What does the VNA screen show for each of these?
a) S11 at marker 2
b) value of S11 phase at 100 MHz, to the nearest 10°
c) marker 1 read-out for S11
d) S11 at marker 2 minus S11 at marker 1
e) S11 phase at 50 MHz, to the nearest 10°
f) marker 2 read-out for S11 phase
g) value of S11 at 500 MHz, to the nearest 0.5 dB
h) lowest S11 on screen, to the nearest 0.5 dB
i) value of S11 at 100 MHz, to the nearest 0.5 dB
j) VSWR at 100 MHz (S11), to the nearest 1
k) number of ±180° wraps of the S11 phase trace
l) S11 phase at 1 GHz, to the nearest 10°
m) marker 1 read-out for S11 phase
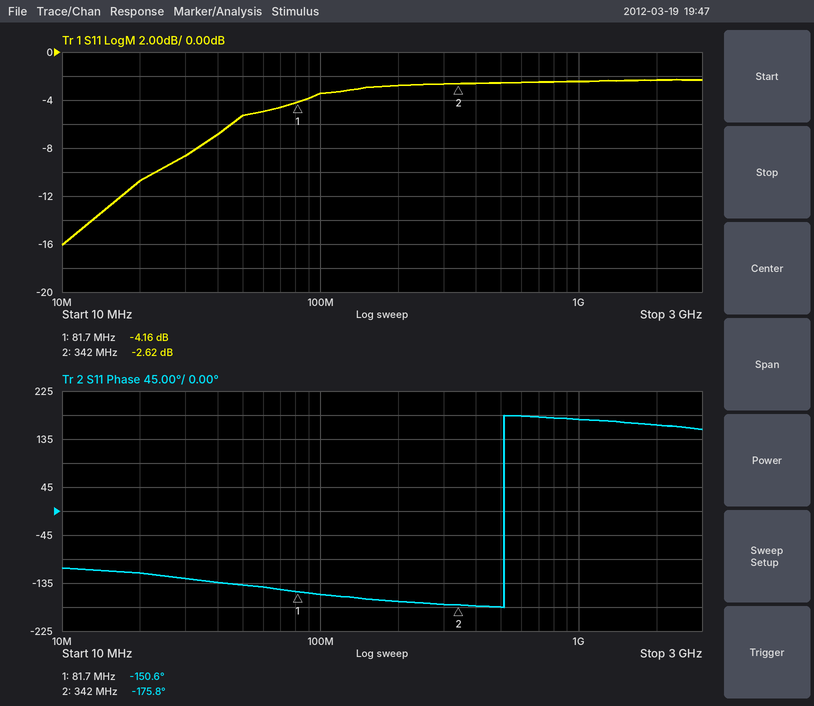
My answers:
-2.62 dB
-160°
-4.16 dB
1.54 dB
-140°
-175.8°
-2.5 dB
-16.0 dB
-3.5 dB
5
1
170°
-150.6°
